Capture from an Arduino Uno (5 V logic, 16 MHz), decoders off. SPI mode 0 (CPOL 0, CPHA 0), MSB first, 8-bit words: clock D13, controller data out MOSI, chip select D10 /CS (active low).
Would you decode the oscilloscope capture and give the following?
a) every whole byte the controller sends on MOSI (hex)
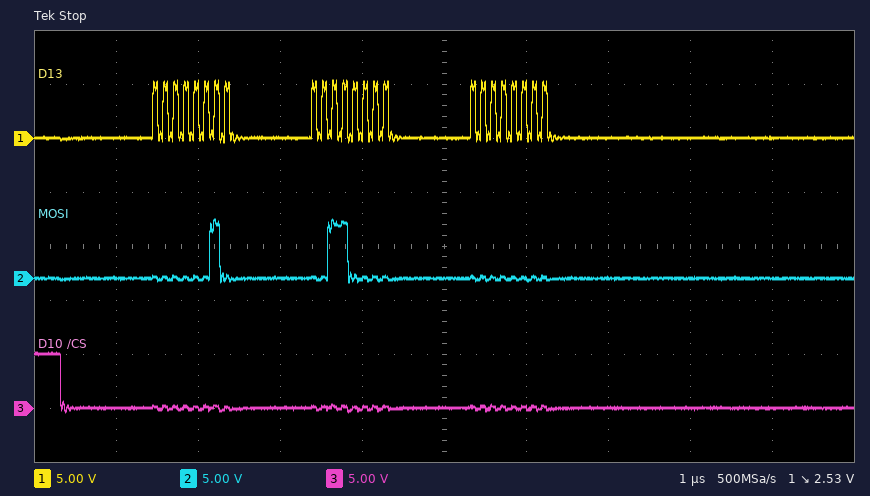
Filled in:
02 30 00
